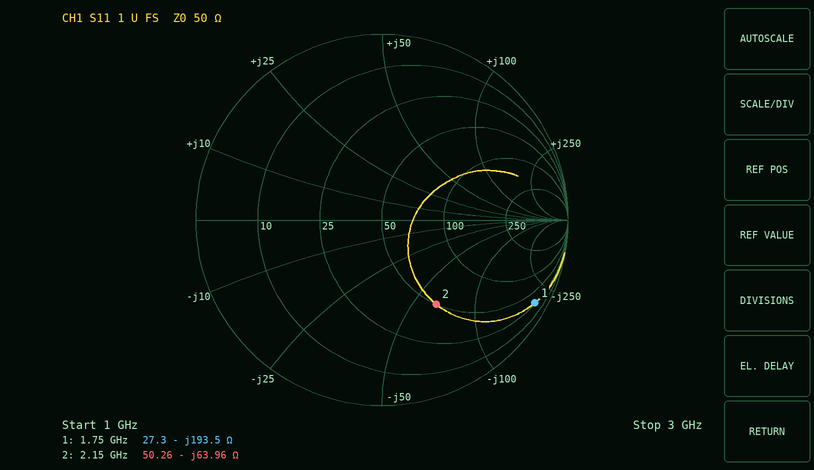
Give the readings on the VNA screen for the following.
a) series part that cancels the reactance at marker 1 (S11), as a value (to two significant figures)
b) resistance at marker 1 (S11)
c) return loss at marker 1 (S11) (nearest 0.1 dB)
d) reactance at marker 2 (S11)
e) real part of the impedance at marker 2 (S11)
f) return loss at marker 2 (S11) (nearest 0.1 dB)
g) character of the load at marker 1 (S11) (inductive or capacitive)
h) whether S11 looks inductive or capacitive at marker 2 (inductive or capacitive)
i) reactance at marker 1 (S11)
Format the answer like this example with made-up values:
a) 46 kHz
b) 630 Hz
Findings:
a) 18 nH
b) 27.3 Ω
c) 0.6 dB
d) -63.96 Ω
e) 50.26 Ω
f) 5.4 dB
g) capacitive
h) capacitive
i) -193.5 Ω
